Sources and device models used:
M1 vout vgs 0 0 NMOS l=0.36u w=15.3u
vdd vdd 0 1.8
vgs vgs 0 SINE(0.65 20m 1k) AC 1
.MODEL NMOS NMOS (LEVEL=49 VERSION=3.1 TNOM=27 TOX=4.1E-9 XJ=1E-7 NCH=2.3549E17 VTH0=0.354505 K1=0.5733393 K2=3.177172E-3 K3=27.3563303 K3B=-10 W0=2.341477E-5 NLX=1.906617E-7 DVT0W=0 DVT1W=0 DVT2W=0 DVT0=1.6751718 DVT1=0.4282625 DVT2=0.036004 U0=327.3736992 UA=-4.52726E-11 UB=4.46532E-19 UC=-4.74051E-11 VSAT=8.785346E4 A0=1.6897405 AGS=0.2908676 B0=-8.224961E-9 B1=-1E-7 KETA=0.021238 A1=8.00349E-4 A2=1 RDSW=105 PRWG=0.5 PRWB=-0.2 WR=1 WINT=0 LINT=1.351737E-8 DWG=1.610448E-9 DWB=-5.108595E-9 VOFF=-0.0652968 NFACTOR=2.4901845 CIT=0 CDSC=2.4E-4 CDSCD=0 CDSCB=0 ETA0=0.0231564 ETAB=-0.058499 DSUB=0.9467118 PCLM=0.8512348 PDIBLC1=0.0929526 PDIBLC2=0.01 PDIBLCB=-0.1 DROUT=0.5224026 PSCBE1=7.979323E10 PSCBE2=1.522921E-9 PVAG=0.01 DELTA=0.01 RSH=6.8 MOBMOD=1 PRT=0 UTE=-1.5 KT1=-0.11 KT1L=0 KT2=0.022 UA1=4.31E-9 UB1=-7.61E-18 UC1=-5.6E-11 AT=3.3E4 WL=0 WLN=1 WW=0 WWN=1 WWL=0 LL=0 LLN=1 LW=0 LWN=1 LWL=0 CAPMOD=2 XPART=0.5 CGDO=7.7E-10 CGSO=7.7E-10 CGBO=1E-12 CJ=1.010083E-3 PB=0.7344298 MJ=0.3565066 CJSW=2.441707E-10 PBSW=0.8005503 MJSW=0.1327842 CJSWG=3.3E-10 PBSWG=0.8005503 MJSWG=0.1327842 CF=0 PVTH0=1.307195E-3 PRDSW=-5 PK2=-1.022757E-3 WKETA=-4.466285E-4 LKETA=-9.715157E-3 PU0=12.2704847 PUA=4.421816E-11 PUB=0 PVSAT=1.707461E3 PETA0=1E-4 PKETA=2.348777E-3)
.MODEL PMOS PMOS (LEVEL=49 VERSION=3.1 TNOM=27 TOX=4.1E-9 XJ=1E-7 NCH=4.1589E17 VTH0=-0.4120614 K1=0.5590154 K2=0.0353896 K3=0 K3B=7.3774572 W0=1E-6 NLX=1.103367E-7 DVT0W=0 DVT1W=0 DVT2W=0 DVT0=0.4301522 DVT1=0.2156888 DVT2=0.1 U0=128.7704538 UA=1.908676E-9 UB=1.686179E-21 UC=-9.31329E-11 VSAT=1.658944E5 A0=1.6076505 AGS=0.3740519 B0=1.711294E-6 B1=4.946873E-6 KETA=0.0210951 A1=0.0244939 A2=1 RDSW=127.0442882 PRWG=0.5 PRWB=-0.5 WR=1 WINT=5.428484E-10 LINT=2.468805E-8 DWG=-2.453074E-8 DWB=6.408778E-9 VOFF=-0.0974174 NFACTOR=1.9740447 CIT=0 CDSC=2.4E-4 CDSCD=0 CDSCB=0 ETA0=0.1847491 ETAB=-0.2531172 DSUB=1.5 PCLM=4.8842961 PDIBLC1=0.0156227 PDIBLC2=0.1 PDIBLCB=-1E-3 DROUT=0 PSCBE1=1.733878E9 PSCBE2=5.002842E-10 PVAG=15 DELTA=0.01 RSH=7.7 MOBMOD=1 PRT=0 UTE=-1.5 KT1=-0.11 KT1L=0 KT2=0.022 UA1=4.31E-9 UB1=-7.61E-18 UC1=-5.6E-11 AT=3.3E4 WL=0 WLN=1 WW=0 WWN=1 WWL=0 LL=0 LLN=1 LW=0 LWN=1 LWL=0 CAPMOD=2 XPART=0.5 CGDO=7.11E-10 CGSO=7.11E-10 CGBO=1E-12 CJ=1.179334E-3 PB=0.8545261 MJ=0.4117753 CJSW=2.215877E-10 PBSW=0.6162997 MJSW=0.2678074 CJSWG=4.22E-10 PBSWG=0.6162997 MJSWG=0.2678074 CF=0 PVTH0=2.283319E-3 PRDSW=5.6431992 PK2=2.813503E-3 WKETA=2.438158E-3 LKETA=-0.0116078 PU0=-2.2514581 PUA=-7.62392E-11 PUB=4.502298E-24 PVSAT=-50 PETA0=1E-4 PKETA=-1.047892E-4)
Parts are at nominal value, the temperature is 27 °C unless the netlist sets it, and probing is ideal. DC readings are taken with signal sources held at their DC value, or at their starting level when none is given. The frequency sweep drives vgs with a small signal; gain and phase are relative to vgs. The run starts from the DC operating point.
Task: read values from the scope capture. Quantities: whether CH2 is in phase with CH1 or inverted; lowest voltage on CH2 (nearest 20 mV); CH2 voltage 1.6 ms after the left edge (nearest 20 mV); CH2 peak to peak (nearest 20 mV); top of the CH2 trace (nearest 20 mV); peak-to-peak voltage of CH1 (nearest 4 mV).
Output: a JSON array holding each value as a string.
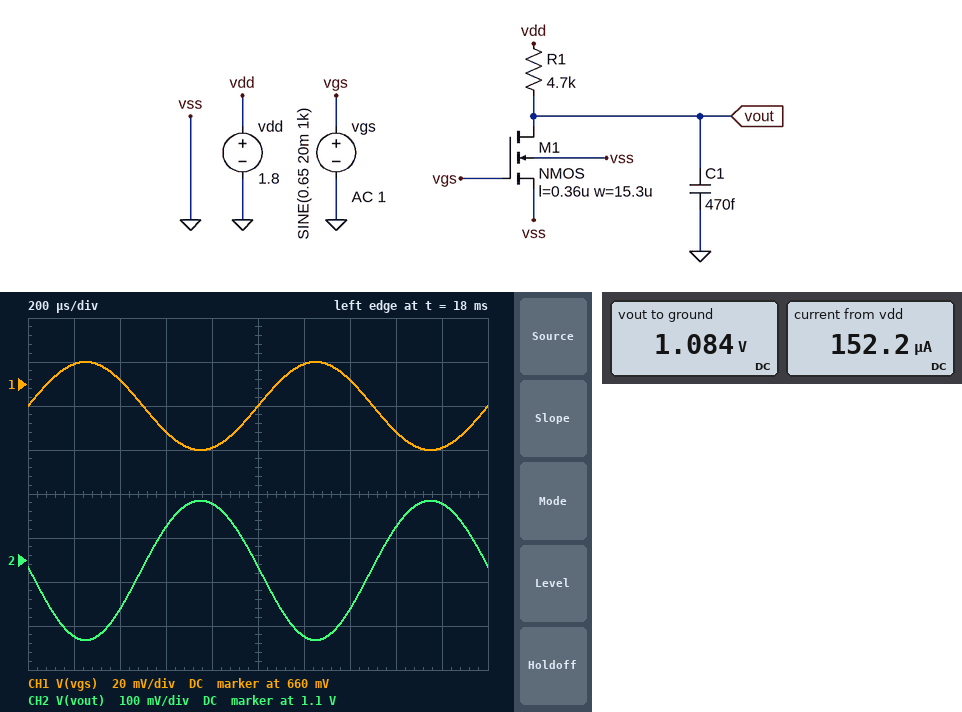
["inverted", "920 mV", "1.18 V", "320 mV", "1.24 V", "40 mV"]
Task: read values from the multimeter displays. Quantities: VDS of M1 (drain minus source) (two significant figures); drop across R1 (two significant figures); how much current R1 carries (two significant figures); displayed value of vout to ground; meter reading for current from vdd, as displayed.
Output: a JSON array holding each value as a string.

["1.1 V", "720 mV", "150 µA", "1.084 V", "152.2 µA"]
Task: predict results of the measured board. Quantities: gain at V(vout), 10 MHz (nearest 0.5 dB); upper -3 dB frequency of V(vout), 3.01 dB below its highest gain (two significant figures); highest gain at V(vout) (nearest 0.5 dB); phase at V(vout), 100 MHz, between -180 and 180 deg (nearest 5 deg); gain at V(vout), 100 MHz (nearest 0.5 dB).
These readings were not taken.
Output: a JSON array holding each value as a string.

["18.0 dB", "75 MHz", "18.0 dB", "125 deg", "13.5 dB"]
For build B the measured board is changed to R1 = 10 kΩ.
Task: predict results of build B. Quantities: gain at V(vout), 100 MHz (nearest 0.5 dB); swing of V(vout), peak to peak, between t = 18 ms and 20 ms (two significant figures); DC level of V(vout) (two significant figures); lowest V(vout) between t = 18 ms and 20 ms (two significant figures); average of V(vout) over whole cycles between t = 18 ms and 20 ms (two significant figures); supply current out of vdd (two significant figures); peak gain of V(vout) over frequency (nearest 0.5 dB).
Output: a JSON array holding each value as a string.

["14.5 dB", "500 mV", "400 mV", "170 mV", "410 mV", "140 µA", "23.0 dB"]
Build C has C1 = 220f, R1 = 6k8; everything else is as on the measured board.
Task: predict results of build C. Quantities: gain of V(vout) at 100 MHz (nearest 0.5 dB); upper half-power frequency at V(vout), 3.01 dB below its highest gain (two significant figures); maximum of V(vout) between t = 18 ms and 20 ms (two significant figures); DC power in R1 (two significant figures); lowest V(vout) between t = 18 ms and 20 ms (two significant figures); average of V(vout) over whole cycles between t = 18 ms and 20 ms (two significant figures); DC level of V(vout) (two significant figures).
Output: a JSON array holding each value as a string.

["18.0 dB", "110 MHz", "1.0 V", "150 µW", "570 mV", "790 mV", "800 mV"]
